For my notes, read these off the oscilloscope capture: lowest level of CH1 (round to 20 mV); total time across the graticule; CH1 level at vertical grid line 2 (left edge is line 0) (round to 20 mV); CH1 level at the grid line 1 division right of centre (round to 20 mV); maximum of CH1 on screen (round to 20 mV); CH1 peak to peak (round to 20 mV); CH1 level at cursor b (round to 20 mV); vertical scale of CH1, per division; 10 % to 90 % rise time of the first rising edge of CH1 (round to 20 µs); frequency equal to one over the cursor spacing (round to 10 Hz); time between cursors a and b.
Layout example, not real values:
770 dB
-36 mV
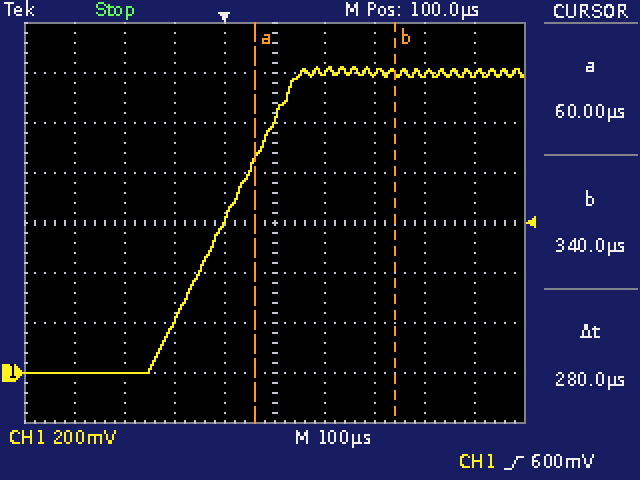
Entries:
0 mV
1 ms
0 mV
1.20 V
1.22 V
1.22 V
1.20 V
200 mV
240 µs
3.57 kHz
280 µs
